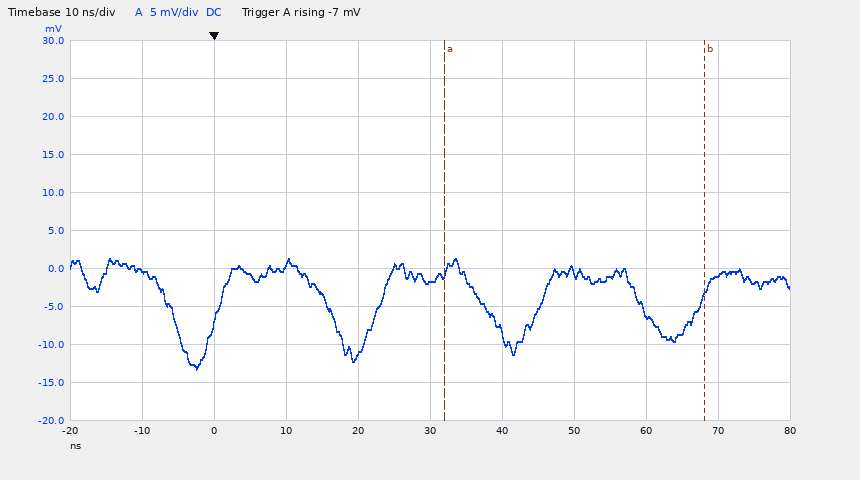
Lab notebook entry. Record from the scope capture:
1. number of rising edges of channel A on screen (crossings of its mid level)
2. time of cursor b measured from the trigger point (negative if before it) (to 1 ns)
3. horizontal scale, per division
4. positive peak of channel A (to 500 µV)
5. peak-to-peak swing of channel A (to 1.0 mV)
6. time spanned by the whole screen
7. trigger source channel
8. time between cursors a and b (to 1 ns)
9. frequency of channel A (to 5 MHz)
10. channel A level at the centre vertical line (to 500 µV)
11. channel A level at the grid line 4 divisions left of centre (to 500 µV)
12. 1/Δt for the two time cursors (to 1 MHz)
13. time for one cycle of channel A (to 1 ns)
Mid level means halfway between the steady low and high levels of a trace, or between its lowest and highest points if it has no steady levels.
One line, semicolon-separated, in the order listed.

4; +68 ns; 10 ns; 1.5 mV; 15.0 mV; 100 ns; channel A; 36 ns; 45 MHz; -2.0 mV; -500 µV; 28 MHz; 22 ns
